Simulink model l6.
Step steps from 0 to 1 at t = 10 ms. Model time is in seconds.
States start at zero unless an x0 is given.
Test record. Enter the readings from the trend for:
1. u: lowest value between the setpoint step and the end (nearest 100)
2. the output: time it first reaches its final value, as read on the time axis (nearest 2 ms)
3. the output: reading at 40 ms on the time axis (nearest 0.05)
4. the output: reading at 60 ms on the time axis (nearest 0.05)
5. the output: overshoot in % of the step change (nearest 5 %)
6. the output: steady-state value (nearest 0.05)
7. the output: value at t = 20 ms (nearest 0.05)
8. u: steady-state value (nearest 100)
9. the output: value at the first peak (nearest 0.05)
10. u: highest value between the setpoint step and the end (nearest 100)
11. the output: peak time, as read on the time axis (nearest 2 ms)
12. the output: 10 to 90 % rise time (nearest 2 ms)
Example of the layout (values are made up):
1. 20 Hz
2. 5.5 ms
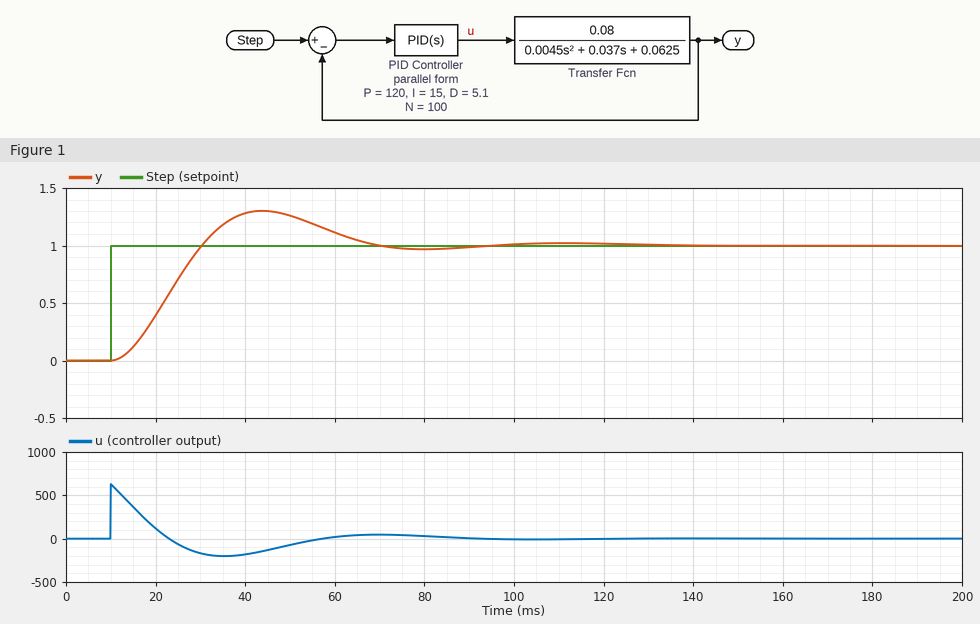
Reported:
1. -200
2. 30 ms
3. 1.30
4. 1.10
5. 30 %
6. 1.00
7. 0.40
8. 0
9. 1.30
10. 600
11. 44 ms
12. 14 ms
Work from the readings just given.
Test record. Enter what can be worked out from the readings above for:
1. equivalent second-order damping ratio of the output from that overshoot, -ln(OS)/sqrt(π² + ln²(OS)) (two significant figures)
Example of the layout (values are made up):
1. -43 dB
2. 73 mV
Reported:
1. 0.36
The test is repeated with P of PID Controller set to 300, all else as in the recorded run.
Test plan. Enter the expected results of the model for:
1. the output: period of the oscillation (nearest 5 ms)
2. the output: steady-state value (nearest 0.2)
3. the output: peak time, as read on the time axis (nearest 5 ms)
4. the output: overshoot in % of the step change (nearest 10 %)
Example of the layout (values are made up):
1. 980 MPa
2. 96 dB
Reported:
1. 60 ms
2. 1.0
3. 40 ms
4. 50 %
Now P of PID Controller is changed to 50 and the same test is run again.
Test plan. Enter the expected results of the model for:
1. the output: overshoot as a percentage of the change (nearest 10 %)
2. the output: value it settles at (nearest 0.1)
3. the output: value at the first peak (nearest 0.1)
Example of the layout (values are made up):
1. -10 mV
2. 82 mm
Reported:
1. 20 %
2. 1.0
3. 1.2
